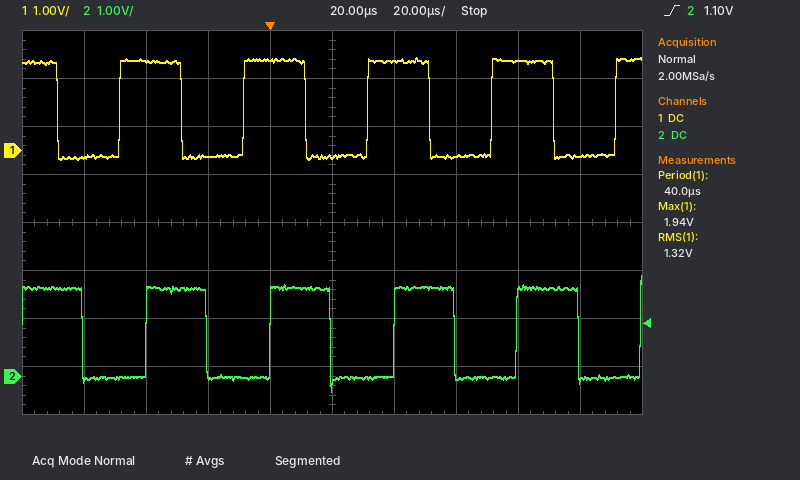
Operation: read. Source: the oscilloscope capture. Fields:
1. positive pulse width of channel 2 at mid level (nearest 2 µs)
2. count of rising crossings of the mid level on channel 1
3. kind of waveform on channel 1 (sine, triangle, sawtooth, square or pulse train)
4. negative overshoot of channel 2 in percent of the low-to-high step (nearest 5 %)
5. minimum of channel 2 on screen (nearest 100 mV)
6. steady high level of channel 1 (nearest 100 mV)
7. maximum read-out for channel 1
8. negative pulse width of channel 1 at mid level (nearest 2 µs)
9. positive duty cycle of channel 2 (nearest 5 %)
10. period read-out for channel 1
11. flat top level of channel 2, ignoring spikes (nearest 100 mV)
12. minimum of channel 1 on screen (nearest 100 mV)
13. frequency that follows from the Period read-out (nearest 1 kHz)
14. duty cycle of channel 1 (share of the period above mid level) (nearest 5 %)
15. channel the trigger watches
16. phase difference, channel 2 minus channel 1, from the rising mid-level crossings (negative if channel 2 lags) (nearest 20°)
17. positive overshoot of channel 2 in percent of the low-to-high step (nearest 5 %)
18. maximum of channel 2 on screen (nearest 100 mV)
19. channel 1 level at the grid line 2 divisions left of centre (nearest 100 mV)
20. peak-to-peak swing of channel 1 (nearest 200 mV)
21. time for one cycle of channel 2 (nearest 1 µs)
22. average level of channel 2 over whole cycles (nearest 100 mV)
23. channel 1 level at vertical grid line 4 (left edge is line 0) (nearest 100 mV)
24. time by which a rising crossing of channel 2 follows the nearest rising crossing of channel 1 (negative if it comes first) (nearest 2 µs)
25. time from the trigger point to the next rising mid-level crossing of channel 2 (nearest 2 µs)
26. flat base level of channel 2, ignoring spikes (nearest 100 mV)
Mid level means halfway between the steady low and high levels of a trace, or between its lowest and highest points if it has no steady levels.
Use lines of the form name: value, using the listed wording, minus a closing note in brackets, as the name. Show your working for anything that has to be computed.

positive pulse width of channel 2 at mid level: 20 µs
count of rising crossings of the mid level on channel 1: 5
kind of waveform on channel 1: square
negative overshoot of channel 2 in percent of the low-to-high step: 15 %
minimum of channel 2 on screen: -300 mV
steady high level of channel 1: 1.9 V
maximum read-out for channel 1: 1.94 V
negative pulse width of channel 1 at mid level: 20 µs
positive duty cycle of channel 2: 20 µs / 40 µs ≈ 50 %
period read-out for channel 1: 40.0 µs
flat top level of channel 2, ignoring spikes: 1.8 V
minimum of channel 1 on screen: -200 mV
frequency that follows from the Period read-out: 1 / 40.0 µs ≈ 25 kHz
duty cycle of channel 1 (share of the period above mid level): 50 %
channel the trigger watches: channel 2
phase difference, channel 2 minus channel 1, from the rising mid-level crossings (negative if channel 2 lags): −360° × (+8 µs) / 40 µs ≈ -72.0°, so -80° to the nearest 20°
positive overshoot of channel 2 in percent of the low-to-high step: 15 %
maximum of channel 2 on screen: 2.1 V
channel 1 level at the grid line 2 divisions left of centre: -100 mV
peak-to-peak swing of channel 1: 2.2 V
time for one cycle of channel 2: 40 µs
average level of channel 2 over whole cycles: 0.0 V + 0.5 × (1.8 V − (0.0 V)) ≈ 900 mV
channel 1 level at vertical grid line 4 (left edge is line 0): 1.9 V
time by which a rising crossing of channel 2 follows the nearest rising crossing of channel 1 (negative if it comes first): +8 µs
time from the trigger point to the next rising mid-level crossing of channel 2: 40 µs
flat base level of channel 2, ignoring spikes: 0.0 V
